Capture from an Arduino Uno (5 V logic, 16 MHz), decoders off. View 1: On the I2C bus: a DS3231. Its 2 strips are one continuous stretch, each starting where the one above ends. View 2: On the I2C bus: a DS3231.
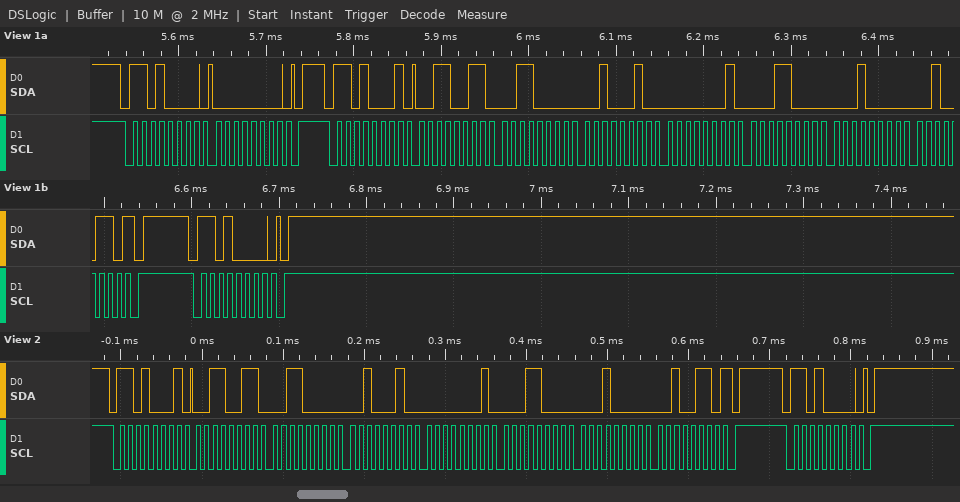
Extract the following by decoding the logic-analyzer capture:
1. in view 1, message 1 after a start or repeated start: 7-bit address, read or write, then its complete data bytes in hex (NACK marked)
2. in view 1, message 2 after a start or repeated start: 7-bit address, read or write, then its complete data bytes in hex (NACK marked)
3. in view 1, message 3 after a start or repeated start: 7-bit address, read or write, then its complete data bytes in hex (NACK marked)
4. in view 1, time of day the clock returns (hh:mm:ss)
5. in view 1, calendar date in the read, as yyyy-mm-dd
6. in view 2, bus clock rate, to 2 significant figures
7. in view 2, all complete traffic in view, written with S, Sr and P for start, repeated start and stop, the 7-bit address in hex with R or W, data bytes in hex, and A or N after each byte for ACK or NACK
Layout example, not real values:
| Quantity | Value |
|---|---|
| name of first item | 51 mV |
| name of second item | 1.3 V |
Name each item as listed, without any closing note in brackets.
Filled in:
| Quantity | Value |
|---|---|
| in view 1, message 1 after a start or repeated start: 7-bit address, read or write, then its complete data bytes in hex | 0x68 write: 00 |
| in view 1, message 2 after a start or repeated start: 7-bit address, read or write, then its complete data bytes in hex | 0x68 read: 33 30 22 01 18 10 26 NACK |
| in view 1, message 3 after a start or repeated start: 7-bit address, read or write, then its complete data bytes in hex | 0x68 write |
| in view 1, time of day the clock returns | 22:30:33 |
| in view 1, calendar date in the read, as yyyy-mm-dd | 2026-10-18 |
| in view 2, bus clock rate, to 2 significant figures | 100 kHz |
| in view 2, all complete traffic in view, written with S, Sr and P for start, repeated start and stop, the 7-bit address in hex with R or W, data bytes in hex, and A or N after each byte for ACK or NACK | S 68R A 33 A 30 A 22 A 01 A 18 A 10 A 26 N P S 68W A P |
